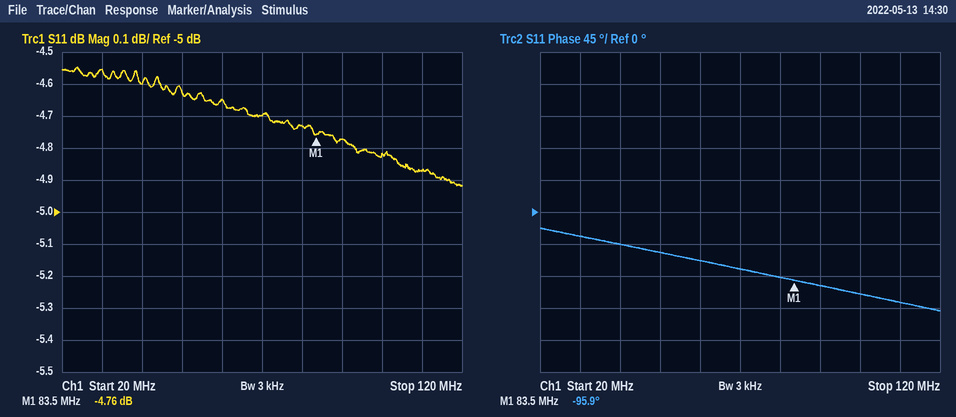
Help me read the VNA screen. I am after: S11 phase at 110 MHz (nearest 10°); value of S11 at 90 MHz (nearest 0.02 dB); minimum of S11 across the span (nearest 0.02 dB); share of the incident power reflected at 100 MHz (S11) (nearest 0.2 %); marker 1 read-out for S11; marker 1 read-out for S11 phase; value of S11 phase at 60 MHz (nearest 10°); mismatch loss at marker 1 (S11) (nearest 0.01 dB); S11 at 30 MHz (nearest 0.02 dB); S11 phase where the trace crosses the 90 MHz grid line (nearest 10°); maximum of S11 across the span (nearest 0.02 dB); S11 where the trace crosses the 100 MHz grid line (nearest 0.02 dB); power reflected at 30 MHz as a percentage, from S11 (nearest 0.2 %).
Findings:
-130°
-4.78 dB
-4.92 dB
33.0 %
-4.76 dB
-95.9°
-70°
1.77 dB
-4.56 dB
-100°
-4.54 dB
-4.82 dB
35.0 %
